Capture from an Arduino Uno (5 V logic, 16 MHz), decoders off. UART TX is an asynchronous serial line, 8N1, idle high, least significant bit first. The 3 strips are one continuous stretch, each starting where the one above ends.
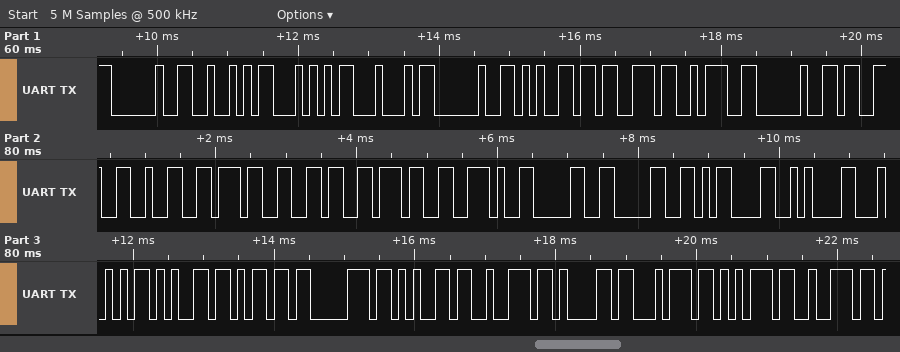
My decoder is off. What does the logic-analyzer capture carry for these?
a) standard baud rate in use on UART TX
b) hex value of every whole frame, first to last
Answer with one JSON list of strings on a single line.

["9600 baud", "20 52 54 44 20 65 73 3A 20 33 32 37 36 37 2E 30 30 0D 0A 54 65 6D 70 65 72 61 74 75 72"]
